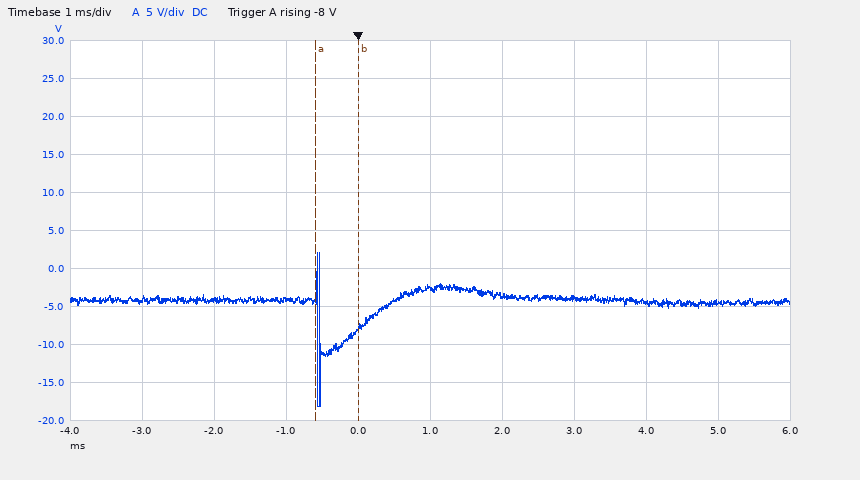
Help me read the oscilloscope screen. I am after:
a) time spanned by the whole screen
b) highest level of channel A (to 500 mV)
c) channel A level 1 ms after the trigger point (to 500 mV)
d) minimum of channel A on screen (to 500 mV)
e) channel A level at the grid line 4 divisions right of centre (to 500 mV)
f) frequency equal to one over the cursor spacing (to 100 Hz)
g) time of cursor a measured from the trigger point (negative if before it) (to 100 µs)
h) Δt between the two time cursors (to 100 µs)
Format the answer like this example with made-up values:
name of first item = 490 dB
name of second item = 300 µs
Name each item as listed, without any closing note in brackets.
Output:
time spanned by the whole screen = 10 ms
highest level of channel A = 2.0 V
channel A level 1 ms after the trigger point = -2.5 V
minimum of channel A on screen = -18.0 V
channel A level at the grid line 4 divisions right of centre = -4.5 V
frequency equal to one over the cursor spacing = 1.7 kHz
time of cursor a measured from the trigger point (negative if before it) = -600 µs
Δt between the two time cursors = 600 µs
